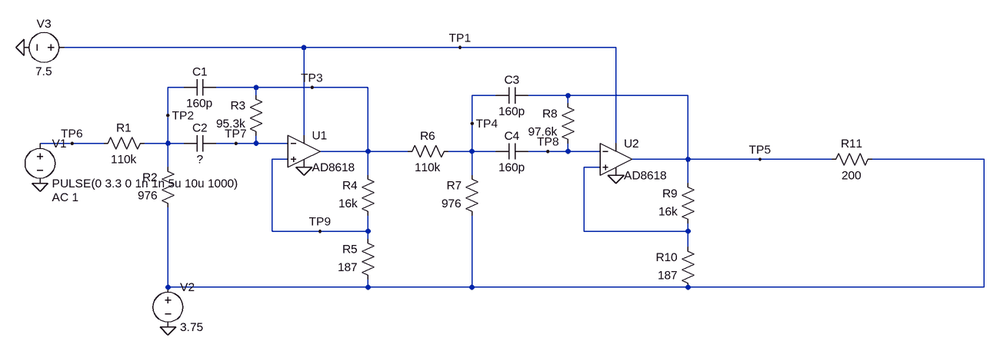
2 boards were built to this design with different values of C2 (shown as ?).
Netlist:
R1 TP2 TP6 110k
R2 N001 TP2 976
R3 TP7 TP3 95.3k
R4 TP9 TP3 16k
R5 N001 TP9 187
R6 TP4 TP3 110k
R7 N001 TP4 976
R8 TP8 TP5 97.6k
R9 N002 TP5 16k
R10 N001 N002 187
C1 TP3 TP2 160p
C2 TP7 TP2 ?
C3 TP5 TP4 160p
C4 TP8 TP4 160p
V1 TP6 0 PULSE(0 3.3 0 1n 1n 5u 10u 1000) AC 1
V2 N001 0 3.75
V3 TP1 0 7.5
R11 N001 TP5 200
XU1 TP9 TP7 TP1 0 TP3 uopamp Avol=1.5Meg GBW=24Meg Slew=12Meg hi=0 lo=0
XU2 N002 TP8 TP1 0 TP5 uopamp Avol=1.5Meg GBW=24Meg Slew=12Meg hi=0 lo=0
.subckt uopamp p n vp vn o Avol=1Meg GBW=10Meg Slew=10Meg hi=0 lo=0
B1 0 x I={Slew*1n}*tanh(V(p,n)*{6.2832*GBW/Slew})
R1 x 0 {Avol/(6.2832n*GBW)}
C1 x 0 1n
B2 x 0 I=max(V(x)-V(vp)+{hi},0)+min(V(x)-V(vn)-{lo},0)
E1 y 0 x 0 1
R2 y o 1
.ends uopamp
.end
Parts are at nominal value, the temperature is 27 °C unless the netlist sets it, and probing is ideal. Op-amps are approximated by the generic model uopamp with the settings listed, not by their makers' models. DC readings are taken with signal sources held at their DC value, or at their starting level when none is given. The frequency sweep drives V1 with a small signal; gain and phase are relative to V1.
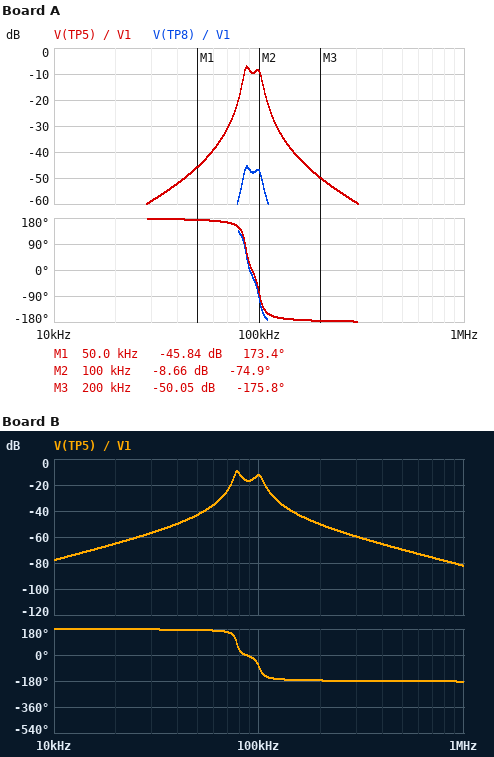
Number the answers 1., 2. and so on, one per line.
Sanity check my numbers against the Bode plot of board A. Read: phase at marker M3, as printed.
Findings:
1. -175.8 deg
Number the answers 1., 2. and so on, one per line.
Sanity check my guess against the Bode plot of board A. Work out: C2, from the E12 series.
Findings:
1. 220 pF
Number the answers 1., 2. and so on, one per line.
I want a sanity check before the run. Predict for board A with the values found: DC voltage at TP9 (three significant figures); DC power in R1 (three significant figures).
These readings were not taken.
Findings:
1. 3.75 V
2. 126 µW
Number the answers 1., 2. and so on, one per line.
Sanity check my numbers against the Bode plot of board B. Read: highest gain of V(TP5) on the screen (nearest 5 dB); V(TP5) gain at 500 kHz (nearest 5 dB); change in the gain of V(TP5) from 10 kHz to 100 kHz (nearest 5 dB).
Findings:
1. -10 dB
2. -70 dB
3. 65 dB
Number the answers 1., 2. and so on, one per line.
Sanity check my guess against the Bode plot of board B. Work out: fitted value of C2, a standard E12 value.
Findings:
1. 270 pF
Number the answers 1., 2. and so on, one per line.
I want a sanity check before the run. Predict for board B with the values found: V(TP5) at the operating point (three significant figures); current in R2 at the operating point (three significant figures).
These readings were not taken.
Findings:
1. 3.75 V
2. 33.8 µA
